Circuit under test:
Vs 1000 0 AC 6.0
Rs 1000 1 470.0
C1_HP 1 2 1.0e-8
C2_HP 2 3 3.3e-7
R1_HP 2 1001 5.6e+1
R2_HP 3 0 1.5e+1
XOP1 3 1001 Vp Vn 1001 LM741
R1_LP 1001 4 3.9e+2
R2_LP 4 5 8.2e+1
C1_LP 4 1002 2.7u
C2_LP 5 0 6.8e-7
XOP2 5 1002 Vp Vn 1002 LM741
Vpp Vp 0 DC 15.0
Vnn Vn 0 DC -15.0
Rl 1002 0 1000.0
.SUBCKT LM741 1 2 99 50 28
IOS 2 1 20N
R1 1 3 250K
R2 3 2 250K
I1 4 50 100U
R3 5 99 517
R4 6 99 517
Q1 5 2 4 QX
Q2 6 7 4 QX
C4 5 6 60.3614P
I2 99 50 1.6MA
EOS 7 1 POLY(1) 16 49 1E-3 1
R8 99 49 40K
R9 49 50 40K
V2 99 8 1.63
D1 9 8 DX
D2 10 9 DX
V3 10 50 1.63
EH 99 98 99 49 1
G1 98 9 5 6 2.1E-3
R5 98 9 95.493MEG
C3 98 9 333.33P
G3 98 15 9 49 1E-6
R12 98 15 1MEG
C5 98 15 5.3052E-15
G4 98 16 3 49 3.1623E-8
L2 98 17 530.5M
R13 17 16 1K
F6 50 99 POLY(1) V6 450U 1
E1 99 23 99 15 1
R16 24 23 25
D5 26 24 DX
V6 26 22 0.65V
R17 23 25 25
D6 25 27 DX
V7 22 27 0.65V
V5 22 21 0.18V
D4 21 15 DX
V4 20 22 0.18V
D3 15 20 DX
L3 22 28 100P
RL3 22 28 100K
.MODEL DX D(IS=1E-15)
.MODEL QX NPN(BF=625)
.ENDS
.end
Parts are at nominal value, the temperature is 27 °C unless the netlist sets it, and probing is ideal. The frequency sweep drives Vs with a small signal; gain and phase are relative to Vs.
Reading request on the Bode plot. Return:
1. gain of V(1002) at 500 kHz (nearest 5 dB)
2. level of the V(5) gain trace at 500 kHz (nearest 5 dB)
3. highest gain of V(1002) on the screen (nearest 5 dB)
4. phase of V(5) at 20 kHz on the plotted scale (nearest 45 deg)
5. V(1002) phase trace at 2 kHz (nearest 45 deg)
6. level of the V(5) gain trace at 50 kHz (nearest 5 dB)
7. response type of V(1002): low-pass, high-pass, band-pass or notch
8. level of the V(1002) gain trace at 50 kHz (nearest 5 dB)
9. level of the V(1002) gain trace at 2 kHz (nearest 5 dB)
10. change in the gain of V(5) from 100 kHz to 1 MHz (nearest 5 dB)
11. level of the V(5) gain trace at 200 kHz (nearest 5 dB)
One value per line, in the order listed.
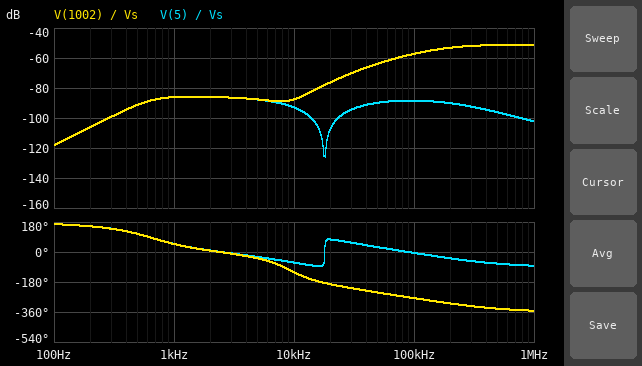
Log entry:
-50 dB
-95 dB
-50 dB
90 deg
0 deg
-90 dB
high-pass
-65 dB
-85 dB
-15 dB
-90 dB
